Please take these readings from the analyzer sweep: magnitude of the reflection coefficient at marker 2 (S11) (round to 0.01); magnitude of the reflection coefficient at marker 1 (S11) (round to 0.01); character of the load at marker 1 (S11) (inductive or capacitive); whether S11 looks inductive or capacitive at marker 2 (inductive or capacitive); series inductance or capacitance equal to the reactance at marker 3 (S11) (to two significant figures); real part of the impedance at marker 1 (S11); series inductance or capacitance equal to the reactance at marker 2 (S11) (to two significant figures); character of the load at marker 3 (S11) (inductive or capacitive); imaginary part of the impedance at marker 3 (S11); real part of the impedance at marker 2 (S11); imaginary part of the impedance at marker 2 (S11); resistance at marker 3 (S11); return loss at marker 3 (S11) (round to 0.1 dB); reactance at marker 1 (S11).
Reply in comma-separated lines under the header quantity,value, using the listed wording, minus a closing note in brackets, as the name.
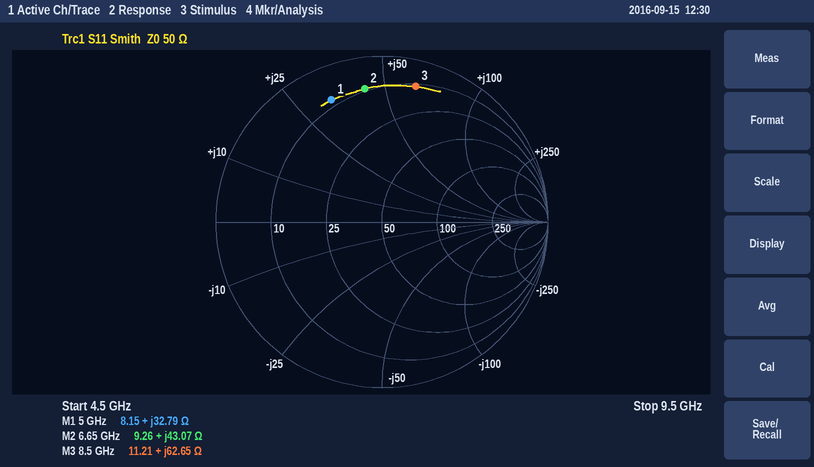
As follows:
quantity,value
magnitude of the reflection coefficient at marker 2 (S11),0.81
magnitude of the reflection coefficient at marker 1 (S11),0.80
character of the load at marker 1 (S11),inductive
whether S11 looks inductive or capacitive at marker 2,inductive
series inductance or capacitance equal to the reactance at marker 3 (S11),1.2 nH
real part of the impedance at marker 1,8.15 Ω
series inductance or capacitance equal to the reactance at marker 2 (S11),1.0 nH
character of the load at marker 3 (S11),inductive
imaginary part of the impedance at marker 3,+62.65 Ω
real part of the impedance at marker 2,9.26 Ω
imaginary part of the impedance at marker 2,+43.07 Ω
resistance at marker 3,11.21 Ω
return loss at marker 3 (S11),1.5 dB
reactance at marker 1,+32.79 Ω
